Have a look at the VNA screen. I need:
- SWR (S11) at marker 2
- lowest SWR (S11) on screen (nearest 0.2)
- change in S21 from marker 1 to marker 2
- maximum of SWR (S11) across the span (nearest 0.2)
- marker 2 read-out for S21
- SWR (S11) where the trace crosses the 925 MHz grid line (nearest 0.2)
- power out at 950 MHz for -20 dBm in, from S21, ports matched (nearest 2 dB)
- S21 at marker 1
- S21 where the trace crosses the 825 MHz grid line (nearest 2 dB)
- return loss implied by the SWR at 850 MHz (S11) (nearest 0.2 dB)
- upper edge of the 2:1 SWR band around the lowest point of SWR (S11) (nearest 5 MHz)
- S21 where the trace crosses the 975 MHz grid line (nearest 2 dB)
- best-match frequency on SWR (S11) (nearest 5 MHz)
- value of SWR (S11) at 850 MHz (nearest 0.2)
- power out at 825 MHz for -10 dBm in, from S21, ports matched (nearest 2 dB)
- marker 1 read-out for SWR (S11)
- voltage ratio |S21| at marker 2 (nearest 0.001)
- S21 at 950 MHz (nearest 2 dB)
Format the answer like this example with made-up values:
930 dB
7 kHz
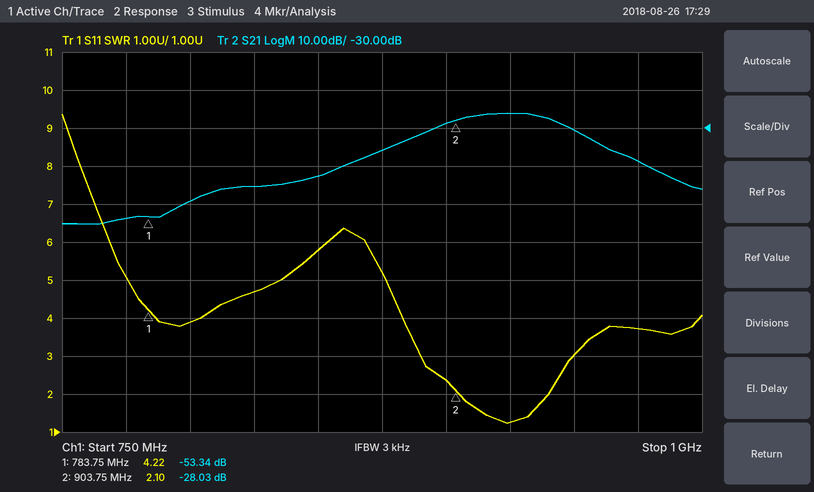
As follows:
2.10
1.2
25.31 dB
9.4
-28.03 dB
1.2
-50 dBm
-53.34 dB
-46 dB
3.0 dB
940 MHz
-38 dB
925 MHz
5.8
-56 dBm
4.22
0.040
-30 dB
